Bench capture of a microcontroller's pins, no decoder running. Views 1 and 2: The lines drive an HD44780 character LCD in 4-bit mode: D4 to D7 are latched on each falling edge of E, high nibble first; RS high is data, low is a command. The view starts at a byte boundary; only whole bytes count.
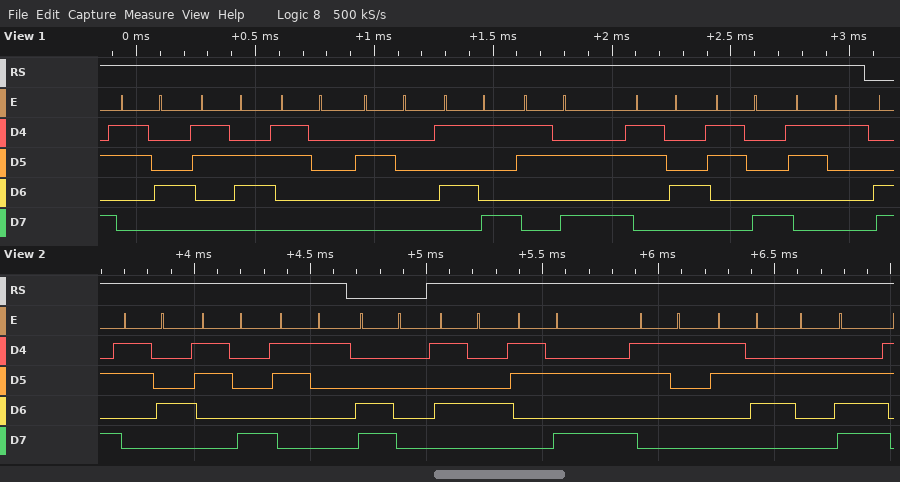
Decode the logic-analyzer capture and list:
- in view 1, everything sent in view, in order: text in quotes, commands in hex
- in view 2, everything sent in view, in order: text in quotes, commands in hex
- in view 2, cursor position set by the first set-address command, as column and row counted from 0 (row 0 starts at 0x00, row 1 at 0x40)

"460 Y:481"
"481" 0xC0 "T:16."
column 0, row 1
